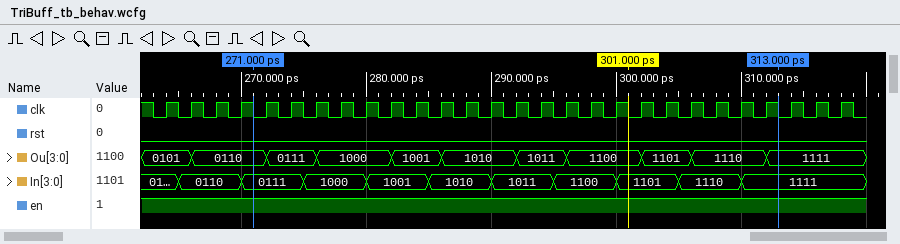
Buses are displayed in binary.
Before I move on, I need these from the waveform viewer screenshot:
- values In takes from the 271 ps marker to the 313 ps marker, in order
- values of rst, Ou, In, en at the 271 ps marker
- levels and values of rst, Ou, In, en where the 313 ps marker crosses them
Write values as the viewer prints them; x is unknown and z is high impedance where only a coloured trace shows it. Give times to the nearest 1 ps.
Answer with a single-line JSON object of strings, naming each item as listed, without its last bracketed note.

{"values In takes from the 271 ps marker to the 313 ps marker, in order": "0111, 1000, 1001, 1010, 1011, 1100, 1101, 1110, 1111", "values of rst, Ou, In, en at the 271 ps marker": "rst=0, Ou=0110, In=0111, en=1", "levels and values of rst, Ou, In, en where the 313 ps marker crosses them": "rst=0, Ou=1111, In=1111, en=1"}
